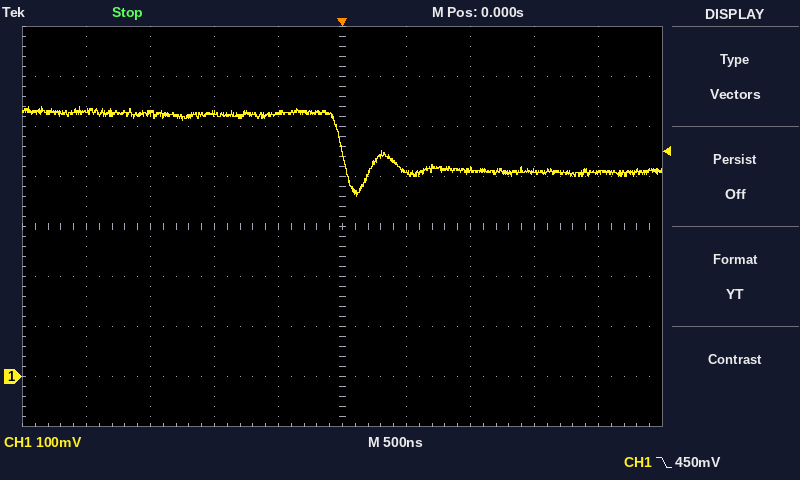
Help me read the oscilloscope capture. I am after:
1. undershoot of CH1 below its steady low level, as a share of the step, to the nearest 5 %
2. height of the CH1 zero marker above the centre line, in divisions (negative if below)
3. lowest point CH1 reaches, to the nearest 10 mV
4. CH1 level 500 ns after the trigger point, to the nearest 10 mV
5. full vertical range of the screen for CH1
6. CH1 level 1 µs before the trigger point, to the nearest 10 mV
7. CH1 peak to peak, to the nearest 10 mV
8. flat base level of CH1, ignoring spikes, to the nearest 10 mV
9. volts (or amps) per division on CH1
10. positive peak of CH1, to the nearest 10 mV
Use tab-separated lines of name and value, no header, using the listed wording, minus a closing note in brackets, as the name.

undershoot of CH1 below its steady low level, as a share of the step, to the nearest 5 %	45 %
height of the CH1 zero marker above the centre line, in divisions	-3.0 div
lowest point CH1 reaches, to the nearest 10 mV	360 mV
CH1 level 500 ns after the trigger point, to the nearest 10 mV	410 mV
full vertical range of the screen for CH1	800 mV
CH1 level 1 µs before the trigger point, to the nearest 10 mV	530 mV
CH1 peak to peak, to the nearest 10 mV	180 mV
flat base level of CH1, ignoring spikes, to the nearest 10 mV	410 mV
volts (or amps) per division on CH1	100 mV
positive peak of CH1, to the nearest 10 mV	540 mV
